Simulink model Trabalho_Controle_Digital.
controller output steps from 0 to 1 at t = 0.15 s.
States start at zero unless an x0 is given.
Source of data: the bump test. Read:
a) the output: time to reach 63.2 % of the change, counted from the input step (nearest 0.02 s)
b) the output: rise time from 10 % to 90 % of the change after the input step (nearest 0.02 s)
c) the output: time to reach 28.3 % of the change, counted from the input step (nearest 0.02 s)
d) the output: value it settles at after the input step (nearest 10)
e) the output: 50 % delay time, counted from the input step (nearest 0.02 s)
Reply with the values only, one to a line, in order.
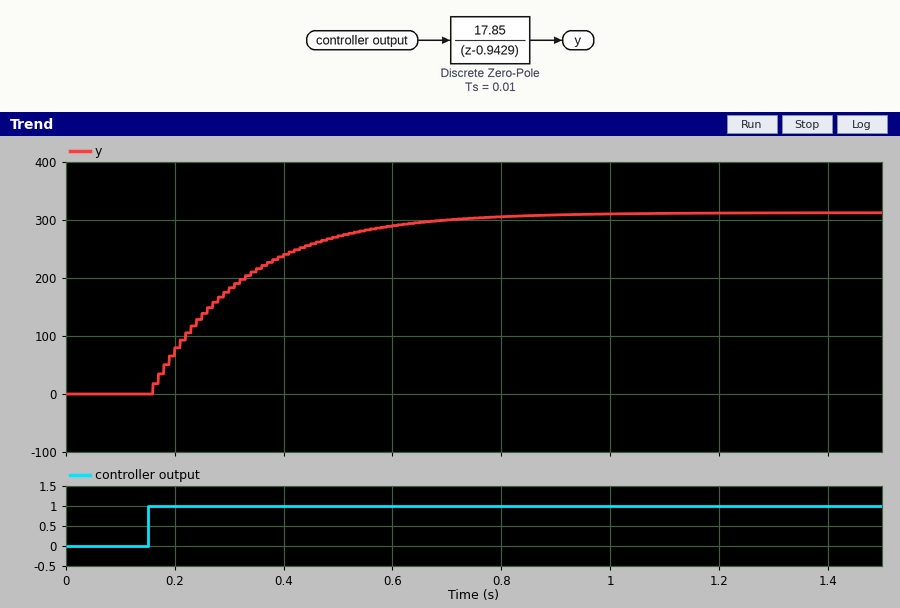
0.18 s
0.38 s
0.06 s
310
0.12 s
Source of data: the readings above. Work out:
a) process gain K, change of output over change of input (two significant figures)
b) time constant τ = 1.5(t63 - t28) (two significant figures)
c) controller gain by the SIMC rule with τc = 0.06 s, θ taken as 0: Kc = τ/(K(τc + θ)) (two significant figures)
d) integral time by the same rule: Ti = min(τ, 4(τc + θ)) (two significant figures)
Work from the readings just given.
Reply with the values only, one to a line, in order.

310
0.18 s
0.0097
0.18 s
